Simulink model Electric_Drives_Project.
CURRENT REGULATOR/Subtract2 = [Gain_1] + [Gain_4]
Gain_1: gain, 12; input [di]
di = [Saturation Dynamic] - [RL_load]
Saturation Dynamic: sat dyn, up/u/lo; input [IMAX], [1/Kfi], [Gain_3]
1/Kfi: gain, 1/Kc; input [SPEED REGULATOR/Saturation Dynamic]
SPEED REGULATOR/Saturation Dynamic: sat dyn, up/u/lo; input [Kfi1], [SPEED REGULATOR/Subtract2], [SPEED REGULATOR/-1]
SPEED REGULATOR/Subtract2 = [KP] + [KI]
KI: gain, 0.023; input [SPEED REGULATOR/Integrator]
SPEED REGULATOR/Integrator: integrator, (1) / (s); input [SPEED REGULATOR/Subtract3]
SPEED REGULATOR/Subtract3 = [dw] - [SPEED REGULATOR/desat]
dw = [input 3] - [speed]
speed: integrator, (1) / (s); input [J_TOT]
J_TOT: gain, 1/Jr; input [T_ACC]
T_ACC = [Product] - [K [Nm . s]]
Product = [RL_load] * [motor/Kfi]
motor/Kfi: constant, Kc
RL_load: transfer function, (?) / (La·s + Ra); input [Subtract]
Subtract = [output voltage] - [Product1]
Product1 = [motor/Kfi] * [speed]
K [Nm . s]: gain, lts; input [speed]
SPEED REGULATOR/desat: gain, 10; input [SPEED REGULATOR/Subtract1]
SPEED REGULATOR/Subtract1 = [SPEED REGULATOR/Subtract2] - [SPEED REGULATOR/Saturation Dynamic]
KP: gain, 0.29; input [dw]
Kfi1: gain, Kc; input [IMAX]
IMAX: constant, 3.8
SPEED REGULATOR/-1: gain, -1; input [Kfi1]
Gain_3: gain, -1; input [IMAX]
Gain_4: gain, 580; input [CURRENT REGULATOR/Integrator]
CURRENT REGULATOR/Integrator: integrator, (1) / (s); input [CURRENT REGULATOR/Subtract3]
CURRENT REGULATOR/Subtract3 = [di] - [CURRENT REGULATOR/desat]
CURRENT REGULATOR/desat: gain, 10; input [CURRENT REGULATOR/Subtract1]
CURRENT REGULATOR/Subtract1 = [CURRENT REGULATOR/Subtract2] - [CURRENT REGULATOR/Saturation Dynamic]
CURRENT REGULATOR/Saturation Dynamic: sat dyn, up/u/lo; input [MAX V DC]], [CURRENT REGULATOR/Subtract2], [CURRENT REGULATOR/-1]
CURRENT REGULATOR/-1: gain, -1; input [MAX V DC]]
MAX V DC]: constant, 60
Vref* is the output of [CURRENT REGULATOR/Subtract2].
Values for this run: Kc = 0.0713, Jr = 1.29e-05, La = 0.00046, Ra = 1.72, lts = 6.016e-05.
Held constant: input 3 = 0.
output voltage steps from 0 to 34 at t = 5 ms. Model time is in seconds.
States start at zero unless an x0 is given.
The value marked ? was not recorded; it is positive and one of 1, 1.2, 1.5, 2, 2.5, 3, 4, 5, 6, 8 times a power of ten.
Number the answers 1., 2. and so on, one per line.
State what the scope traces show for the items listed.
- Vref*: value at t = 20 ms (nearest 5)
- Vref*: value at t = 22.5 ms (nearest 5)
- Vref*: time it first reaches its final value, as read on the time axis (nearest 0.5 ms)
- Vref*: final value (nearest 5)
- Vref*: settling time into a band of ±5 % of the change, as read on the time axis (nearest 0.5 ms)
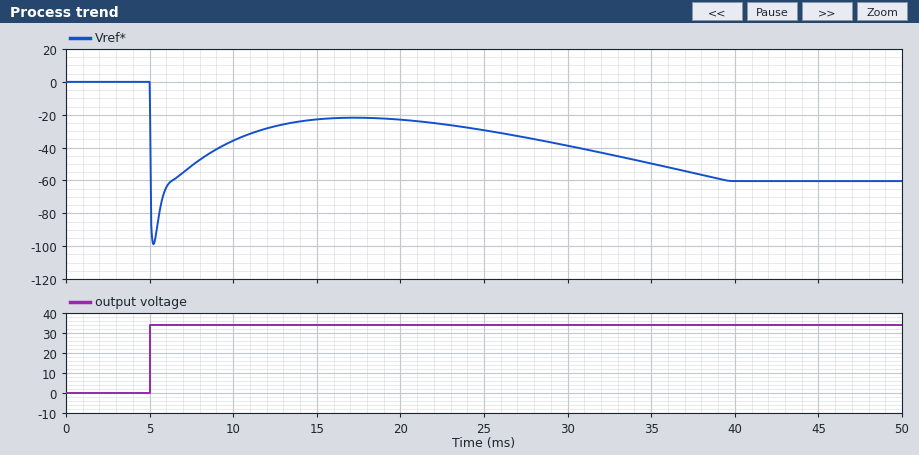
1. -25
2. -25
3. 5.0 ms
4. -60
5. 38.5 ms
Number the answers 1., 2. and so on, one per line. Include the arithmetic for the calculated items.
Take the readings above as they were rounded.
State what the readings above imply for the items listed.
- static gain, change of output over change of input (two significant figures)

1. (-60 - 0) / (34 - 0) = -1.8
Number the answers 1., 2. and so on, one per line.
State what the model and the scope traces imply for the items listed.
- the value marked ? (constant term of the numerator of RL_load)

1. 0.6
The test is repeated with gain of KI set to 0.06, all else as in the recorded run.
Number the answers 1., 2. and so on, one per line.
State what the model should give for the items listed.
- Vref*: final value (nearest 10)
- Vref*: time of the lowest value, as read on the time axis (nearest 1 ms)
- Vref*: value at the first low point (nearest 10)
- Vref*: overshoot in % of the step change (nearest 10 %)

1. -60
2. 5 ms
3. -100
4. 60 %
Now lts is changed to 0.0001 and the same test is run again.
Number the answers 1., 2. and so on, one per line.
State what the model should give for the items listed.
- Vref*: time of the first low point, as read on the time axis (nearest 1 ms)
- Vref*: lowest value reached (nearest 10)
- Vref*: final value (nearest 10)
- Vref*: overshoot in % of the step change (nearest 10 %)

1. 5 ms
2. -100
3. -60
4. 60 %
